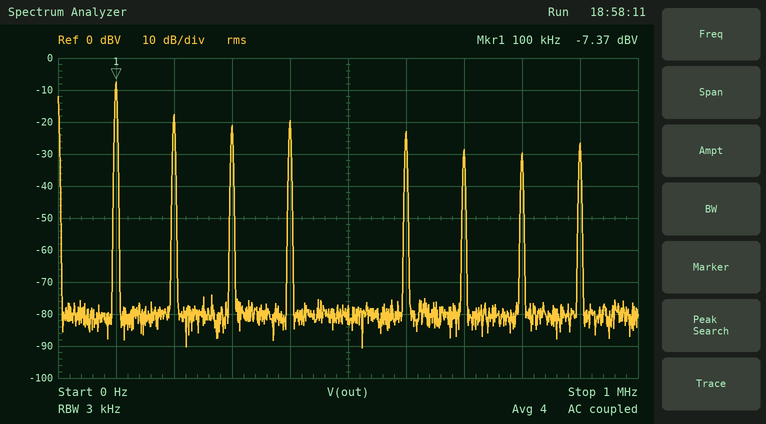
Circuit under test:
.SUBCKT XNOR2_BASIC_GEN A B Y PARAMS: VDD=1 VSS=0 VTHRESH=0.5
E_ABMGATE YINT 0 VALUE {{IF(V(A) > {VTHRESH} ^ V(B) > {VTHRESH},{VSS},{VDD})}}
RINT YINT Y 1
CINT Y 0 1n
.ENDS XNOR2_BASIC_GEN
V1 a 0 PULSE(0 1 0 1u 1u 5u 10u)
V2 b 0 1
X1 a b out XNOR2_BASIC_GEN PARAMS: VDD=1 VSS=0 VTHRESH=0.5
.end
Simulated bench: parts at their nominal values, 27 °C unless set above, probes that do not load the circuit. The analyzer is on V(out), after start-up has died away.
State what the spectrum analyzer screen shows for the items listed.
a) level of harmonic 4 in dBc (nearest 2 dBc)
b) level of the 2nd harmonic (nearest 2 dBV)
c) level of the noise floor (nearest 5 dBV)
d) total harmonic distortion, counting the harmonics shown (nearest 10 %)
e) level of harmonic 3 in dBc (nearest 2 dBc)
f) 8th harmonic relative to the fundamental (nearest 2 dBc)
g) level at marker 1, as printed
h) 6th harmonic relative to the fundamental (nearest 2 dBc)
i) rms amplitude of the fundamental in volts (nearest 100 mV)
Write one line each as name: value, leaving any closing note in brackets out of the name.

level of harmonic 4 in dBc: -12 dBc
level of the 2nd harmonic: -18 dBV
level of the noise floor: -80 dBV
total harmonic distortion, counting the harmonics shown: 50 %
level of harmonic 3 in dBc: -14 dBc
8th harmonic relative to the fundamental: -22 dBc
level at marker 1, as printed: -7.37 dBV
6th harmonic relative to the fundamental: -16 dBc
rms amplitude of the fundamental in volts: 400 mV
